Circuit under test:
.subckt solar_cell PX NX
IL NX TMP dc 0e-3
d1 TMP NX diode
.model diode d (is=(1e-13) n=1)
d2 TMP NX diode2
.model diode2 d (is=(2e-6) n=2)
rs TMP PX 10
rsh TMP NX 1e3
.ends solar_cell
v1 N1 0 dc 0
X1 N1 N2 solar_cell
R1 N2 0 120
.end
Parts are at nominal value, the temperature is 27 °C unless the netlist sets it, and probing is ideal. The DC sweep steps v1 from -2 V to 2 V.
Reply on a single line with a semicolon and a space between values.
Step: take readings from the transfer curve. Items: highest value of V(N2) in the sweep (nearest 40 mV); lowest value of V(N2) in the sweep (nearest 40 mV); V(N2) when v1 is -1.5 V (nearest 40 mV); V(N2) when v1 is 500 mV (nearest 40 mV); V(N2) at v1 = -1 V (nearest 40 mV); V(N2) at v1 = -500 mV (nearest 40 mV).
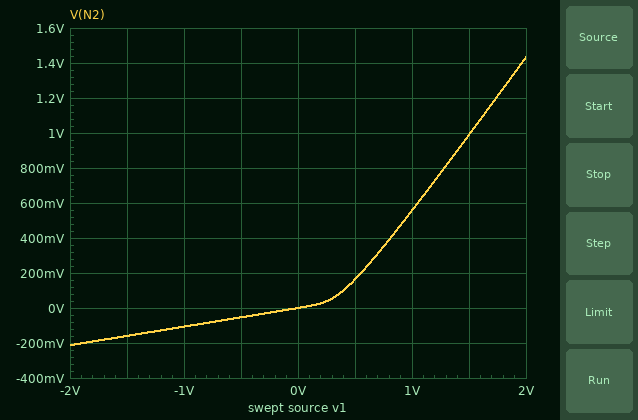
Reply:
1.44 V; -200 mV; -160 mV; 160 mV; -120 mV; -40 mV
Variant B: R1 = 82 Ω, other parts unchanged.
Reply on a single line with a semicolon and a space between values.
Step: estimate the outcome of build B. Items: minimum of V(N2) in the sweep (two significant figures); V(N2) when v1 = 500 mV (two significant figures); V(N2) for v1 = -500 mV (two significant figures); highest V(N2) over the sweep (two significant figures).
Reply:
-150 mV; 140 mV; -38 mV; 1.4 V
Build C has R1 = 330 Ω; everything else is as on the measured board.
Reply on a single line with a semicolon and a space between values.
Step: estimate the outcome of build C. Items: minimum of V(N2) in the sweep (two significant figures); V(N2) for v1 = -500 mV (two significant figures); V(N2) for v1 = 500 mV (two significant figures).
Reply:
-490 mV; -120 mV; 220 mV
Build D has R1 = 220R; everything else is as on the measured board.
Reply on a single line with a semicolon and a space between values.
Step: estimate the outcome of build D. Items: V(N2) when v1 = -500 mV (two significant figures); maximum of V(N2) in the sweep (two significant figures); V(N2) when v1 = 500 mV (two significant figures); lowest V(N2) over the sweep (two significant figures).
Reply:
-90 mV; 1.5 V; 200 mV; -360 mV
